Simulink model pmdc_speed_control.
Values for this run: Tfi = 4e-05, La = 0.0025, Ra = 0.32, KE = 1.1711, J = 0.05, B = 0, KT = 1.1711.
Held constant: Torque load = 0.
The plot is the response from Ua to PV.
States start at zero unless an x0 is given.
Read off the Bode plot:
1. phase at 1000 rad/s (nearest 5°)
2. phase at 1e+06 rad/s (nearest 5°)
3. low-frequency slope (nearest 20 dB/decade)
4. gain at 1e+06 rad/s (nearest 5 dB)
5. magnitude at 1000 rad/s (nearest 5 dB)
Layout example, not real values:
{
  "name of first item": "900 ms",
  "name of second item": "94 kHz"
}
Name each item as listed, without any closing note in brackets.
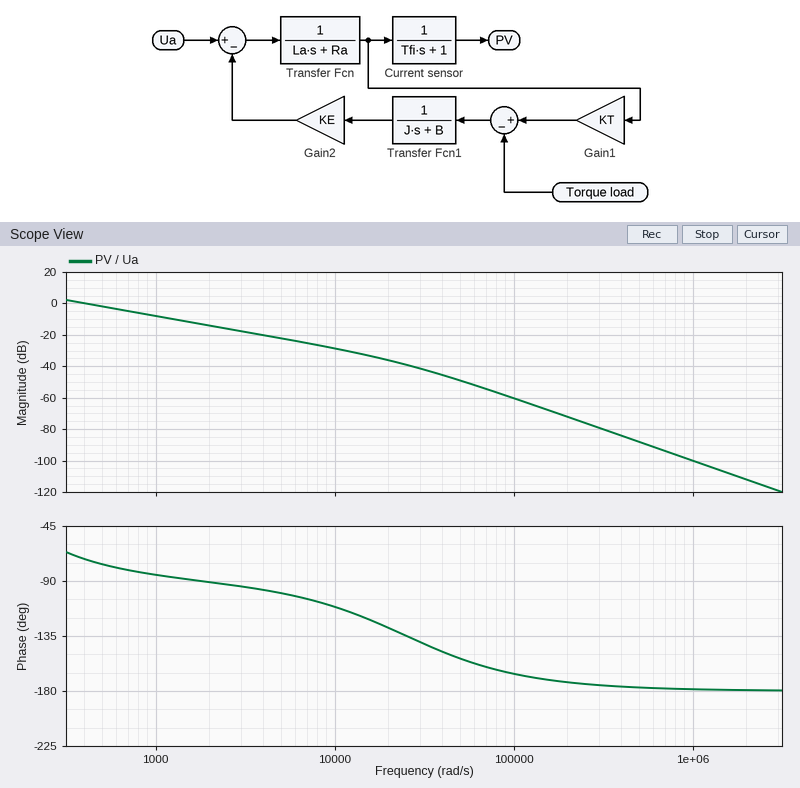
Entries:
{
  "phase at 1000 rad/s": "-85°",
  "phase at 1e+06 rad/s": "-180°",
  "low-frequency slope": "-20 dB/decade",
  "gain at 1e+06 rad/s": "-100 dB",
  "magnitude at 1000 rad/s": "-10 dB"
}
